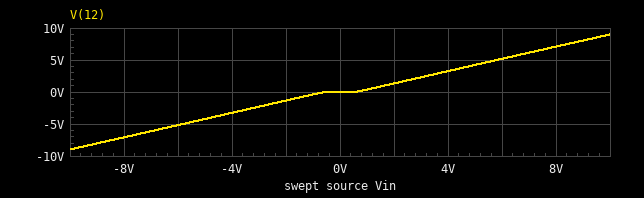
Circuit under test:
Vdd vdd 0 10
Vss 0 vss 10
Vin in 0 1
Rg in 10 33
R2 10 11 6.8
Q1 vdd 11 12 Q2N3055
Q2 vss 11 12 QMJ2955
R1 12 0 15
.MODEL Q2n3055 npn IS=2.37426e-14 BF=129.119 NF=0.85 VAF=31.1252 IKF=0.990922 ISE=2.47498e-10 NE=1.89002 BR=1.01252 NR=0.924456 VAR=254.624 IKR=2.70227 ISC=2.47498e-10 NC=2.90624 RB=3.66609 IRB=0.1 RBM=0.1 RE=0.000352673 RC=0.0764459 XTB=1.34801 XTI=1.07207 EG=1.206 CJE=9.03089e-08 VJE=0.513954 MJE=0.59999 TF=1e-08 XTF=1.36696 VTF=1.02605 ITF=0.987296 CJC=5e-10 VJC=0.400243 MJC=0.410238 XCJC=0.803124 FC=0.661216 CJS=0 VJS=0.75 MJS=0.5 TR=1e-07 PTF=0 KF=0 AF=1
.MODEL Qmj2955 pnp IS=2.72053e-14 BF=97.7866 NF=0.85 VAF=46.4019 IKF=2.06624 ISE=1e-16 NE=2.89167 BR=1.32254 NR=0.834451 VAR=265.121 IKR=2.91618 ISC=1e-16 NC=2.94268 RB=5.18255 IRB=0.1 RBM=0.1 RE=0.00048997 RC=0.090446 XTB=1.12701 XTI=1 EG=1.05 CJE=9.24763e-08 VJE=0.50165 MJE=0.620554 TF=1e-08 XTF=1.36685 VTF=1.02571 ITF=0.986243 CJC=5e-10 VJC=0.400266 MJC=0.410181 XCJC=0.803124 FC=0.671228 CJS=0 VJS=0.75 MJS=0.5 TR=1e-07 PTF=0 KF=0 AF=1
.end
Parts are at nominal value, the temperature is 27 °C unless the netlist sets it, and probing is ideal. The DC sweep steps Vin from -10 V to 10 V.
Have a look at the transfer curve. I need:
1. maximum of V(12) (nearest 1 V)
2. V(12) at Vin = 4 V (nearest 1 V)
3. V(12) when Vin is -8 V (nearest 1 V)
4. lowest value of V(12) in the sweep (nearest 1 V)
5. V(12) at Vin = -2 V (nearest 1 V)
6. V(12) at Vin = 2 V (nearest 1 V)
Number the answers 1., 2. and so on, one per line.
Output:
1. 9 V
2. 3 V
3. -7 V
4. -9 V
5. -1 V
6. 1 V
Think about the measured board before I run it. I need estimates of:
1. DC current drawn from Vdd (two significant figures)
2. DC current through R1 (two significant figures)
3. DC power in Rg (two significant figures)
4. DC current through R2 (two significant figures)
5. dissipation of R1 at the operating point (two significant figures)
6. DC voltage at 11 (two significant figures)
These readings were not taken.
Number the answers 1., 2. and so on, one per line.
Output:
1. 26 mA
2. 26 mA
3. 1.5 µW
4. 210 µA
5. 10 mW
6. 990 mV
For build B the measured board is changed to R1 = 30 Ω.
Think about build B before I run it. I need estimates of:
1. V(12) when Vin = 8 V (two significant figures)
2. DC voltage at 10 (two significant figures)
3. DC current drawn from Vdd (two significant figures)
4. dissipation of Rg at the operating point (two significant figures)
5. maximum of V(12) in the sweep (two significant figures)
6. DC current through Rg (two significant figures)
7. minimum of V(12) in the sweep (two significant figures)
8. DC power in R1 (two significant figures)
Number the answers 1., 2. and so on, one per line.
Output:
1. 7.2 V
2. 1.0 V
3. 13 mA
4. 510 nW
5. 9.2 V
6. 120 µA
7. -9.2 V
8. 5.5 mW
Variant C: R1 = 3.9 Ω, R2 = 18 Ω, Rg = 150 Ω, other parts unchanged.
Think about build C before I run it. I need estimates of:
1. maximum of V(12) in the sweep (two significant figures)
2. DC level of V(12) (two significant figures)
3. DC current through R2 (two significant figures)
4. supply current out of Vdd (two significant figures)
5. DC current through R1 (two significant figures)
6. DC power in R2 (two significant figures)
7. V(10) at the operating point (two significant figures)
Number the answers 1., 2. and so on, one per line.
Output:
1. 5.5 V
2. 280 mV
3. 540 µA
4. 71 mA
5. 72 mA
6. 5.3 µW
7. 920 mV
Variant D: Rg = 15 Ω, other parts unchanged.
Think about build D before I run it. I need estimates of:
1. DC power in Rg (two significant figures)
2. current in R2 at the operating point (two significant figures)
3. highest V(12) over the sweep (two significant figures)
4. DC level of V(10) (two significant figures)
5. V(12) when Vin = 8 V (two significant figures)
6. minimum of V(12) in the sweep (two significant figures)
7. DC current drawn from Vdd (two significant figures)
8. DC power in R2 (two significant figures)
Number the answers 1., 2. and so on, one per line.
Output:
1. 700 nW
2. 220 µA
3. 9.1 V
4. 1.0 V
5. 7.2 V
6. -9.1 V
7. 26 mA
8. 320 nW
